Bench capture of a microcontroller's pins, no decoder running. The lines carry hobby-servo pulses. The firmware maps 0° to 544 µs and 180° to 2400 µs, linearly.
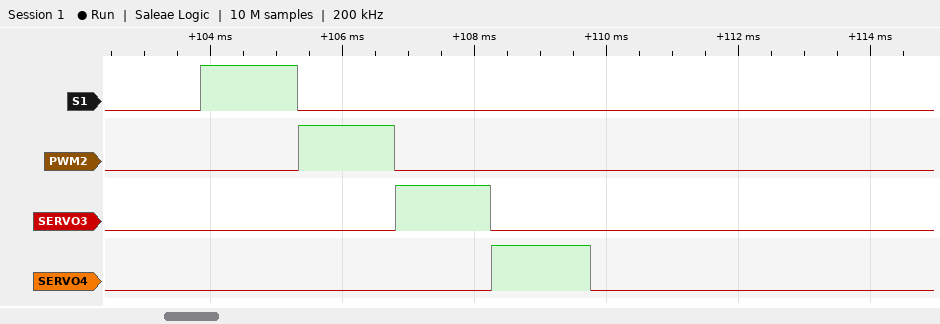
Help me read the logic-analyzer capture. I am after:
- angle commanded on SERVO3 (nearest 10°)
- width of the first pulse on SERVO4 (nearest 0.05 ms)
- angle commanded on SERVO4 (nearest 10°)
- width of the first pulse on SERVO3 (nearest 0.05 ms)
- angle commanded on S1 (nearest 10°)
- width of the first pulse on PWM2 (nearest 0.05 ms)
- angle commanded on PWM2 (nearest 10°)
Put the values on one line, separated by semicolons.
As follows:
90°; 1.50 ms; 90°; 1.45 ms; 90°; 1.45 ms; 90°
